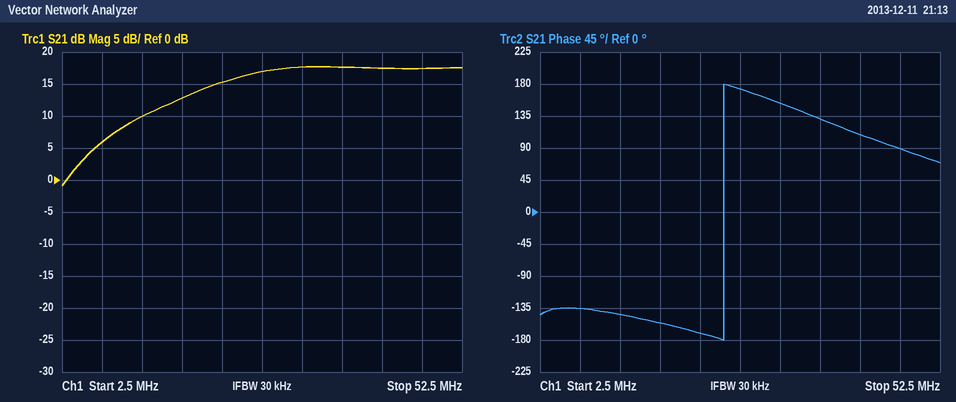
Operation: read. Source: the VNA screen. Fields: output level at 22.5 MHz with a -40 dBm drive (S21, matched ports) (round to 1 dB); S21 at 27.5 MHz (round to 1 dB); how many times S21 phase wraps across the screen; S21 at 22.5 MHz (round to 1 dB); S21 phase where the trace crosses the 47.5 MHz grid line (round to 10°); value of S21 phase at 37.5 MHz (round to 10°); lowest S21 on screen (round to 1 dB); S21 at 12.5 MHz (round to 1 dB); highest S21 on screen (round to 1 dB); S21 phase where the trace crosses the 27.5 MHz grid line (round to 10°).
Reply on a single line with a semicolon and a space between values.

-25 dBm; 17 dB; 1; 15 dB; 90°; 130°; -1 dB; 10 dB; 18 dB; 170°
